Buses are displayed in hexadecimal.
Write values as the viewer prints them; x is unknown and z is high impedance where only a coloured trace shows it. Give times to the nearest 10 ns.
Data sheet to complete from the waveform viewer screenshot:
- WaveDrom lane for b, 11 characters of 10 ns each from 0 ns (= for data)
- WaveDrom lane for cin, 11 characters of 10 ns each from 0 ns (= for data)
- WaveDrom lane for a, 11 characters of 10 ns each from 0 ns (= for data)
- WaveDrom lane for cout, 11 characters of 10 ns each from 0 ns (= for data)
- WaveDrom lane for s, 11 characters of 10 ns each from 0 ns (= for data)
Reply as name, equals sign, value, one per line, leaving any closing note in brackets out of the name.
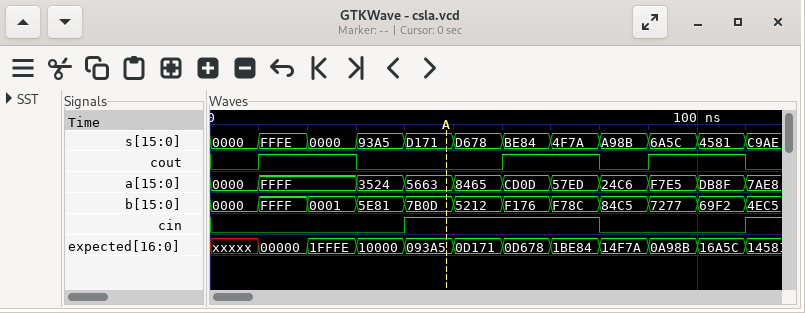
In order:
WaveDrom lane for b, 11 characters of 10 ns each from 0 ns = {name: 'b', wave: '===========', data: '0000 FFFF 0001 5E81 7B0D 5212 F176 F78C 84C5 7277 69F2'}
WaveDrom lane for cin, 11 characters of 10 ns each from 0 ns = {name: 'cin', wave: '0...1...0..'}
WaveDrom lane for a, 11 characters of 10 ns each from 0 ns = {name: 'a', wave: '==.========', data: '0000 FFFF 3524 5663 8465 CD0D 57ED 24C6 F7E5 DB8F'}
WaveDrom lane for cout, 11 characters of 10 ns each from 0 ns = {name: 'cout', wave: '01.0..1.01.'}
WaveDrom lane for s, 11 characters of 10 ns each from 0 ns = {name: 's', wave: '===========', data: '0000 FFFE 0000 93A5 D171 D678 BE84 4F7A A98B 6A5C 4581'}
